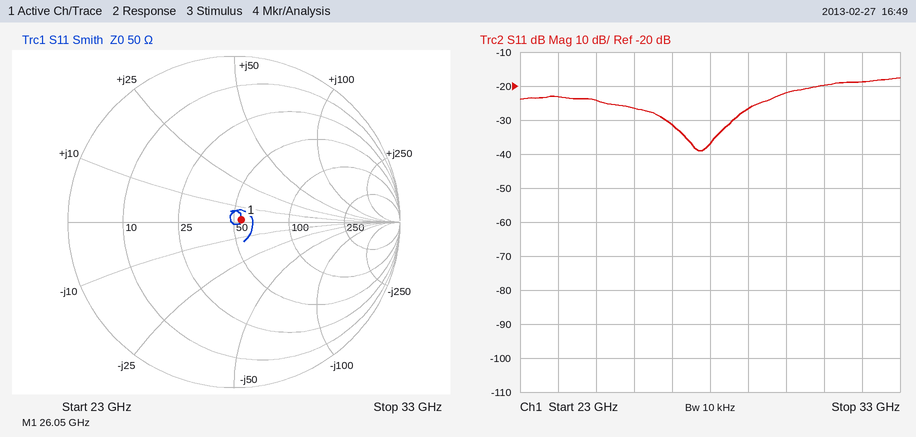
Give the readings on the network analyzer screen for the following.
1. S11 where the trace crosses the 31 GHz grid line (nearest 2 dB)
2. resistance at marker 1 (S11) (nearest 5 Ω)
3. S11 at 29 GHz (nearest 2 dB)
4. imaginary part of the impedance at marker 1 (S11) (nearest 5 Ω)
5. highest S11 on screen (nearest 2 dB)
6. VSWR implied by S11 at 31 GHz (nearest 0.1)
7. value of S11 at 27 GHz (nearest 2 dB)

-20 dB
55 Ω
-26 dB
0 Ω
-18 dB
1.2
-32 dB
